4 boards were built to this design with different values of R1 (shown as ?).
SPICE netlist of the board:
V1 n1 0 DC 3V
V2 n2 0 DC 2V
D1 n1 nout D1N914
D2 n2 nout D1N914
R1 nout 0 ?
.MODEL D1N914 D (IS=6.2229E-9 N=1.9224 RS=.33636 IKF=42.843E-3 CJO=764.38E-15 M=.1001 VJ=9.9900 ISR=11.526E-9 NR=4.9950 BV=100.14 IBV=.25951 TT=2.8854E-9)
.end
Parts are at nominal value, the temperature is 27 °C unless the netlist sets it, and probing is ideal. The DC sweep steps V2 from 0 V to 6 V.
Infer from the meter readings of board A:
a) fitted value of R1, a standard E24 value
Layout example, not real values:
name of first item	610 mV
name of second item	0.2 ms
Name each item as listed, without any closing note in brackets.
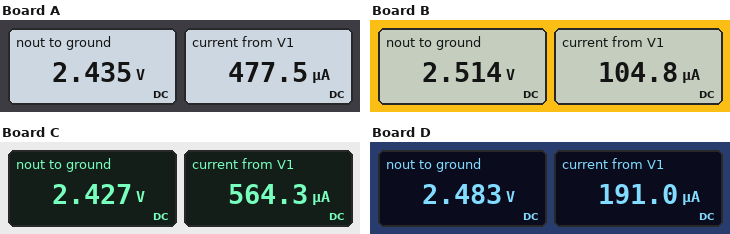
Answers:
fitted value of R1, a standard E24 value	5.1 kΩ
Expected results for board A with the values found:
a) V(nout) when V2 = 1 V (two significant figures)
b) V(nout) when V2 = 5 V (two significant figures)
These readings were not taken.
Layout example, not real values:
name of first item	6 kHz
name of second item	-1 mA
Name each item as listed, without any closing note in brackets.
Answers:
V(nout) when V2 = 1 V	2.4 V
V(nout) when V2 = 5 V	4.4 V
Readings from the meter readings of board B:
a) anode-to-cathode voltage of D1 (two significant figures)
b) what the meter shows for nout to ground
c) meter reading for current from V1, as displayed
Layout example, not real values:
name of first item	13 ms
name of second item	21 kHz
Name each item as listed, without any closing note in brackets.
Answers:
anode-to-cathode voltage of D1	490 mV
what the meter shows for nout to ground	2.514 V
meter reading for current from V1, as displayed	104.8 µA
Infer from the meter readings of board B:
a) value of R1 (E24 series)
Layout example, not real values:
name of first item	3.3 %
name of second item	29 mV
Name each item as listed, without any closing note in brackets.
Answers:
value of R1	24 kΩ
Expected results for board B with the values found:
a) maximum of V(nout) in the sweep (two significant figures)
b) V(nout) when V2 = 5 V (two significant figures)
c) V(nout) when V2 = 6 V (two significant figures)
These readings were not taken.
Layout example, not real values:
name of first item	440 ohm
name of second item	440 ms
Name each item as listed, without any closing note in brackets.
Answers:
maximum of V(nout) in the sweep	5.5 V
V(nout) when V2 = 5 V	4.5 V
V(nout) when V2 = 6 V	5.5 V
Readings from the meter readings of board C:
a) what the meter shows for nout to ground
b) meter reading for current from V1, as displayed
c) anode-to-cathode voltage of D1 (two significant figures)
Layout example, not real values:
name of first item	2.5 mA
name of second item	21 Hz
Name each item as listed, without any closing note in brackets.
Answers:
what the meter shows for nout to ground	2.427 V
meter reading for current from V1, as displayed	564.3 µA
anode-to-cathode voltage of D1	570 mV
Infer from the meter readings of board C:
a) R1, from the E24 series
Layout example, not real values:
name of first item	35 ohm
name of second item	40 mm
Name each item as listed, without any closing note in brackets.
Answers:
R1, from the E24 series	4.3 kΩ
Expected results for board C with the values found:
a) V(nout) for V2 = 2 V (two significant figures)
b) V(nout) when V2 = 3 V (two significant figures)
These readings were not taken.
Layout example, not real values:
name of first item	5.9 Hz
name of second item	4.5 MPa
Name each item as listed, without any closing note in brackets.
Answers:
V(nout) for V2 = 2 V	2.4 V
V(nout) when V2 = 3 V	2.5 V
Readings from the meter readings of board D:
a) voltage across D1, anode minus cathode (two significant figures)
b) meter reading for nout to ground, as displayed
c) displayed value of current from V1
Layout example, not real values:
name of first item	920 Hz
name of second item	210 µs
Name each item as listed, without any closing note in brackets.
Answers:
voltage across D1, anode minus cathode	520 mV
meter reading for nout to ground, as displayed	2.483 V
displayed value of current from V1	191.0 µA
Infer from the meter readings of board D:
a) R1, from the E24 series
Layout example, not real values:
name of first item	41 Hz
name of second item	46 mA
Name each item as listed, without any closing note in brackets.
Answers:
R1, from the E24 series	13 kΩ
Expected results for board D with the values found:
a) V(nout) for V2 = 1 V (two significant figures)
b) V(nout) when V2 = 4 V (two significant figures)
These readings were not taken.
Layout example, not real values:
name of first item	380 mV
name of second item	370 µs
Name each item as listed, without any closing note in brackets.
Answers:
V(nout) for V2 = 1 V	2.5 V
V(nout) when V2 = 4 V	3.5 V
